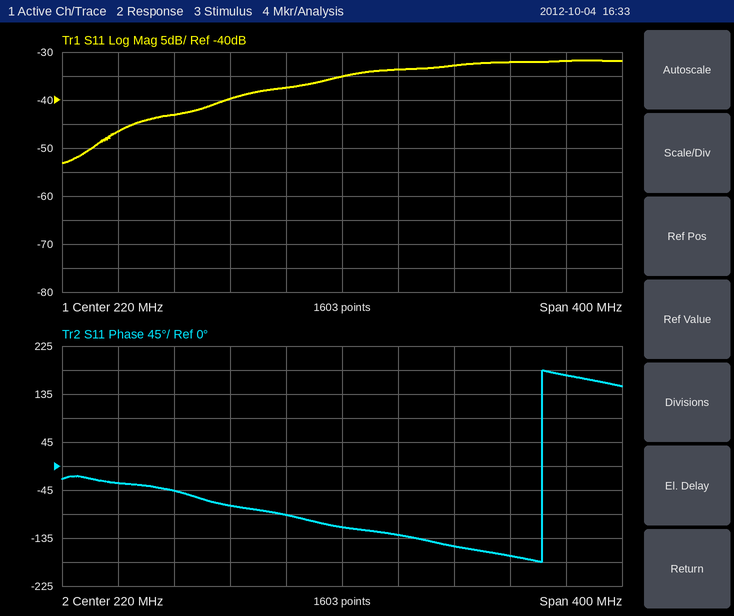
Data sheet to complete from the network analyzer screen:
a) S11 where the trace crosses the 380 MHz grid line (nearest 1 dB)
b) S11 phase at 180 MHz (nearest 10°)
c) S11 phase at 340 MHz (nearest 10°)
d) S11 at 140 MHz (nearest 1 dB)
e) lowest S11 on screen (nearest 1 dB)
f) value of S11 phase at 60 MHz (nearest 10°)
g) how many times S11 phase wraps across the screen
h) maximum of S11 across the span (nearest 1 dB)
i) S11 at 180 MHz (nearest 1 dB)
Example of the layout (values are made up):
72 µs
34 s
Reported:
-32 dB
-90°
-170°
-40 dB
-53 dB
-30°
1
-32 dB
-37 dB
